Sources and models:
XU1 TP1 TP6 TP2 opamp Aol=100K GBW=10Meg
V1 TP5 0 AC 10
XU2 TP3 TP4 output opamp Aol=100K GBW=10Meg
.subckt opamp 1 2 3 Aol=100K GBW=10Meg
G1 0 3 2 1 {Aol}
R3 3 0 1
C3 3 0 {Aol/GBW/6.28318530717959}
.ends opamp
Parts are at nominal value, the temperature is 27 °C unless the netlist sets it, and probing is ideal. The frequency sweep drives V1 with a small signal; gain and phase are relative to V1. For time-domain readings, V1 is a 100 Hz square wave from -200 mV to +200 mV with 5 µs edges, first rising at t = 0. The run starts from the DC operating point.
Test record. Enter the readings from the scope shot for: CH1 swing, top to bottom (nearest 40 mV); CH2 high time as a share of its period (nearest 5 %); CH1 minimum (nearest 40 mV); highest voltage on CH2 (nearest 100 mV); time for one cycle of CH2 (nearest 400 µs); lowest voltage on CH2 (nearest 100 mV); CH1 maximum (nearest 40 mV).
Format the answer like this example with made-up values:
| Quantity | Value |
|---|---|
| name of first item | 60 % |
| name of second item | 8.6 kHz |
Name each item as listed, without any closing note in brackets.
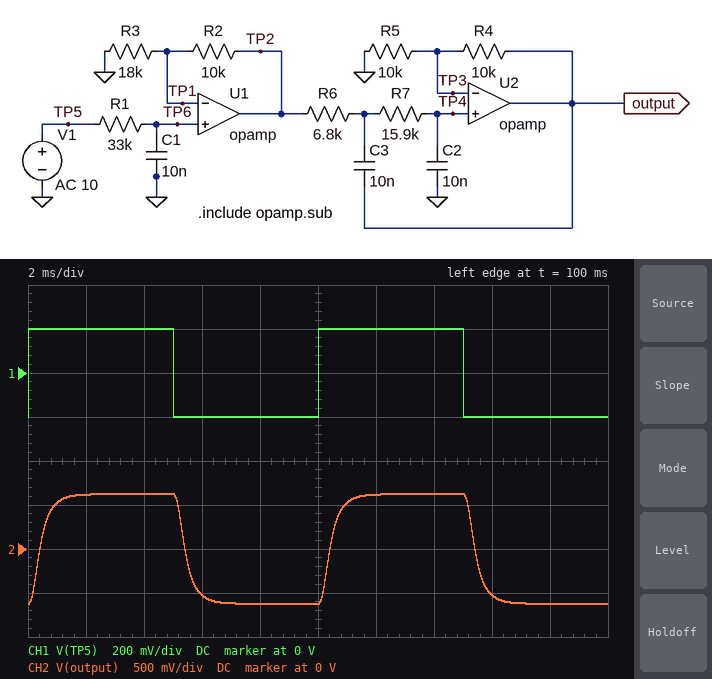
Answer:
| Quantity | Value |
|---|---|
| CH1 swing, top to bottom | 400 mV |
| CH2 high time as a share of its period | 50 % |
| CH1 minimum | -200 mV |
| highest voltage on CH2 | 600 mV |
| time for one cycle of CH2 | 10.0 ms |
| lowest voltage on CH2 | -600 mV |
| CH1 maximum | 200 mV |
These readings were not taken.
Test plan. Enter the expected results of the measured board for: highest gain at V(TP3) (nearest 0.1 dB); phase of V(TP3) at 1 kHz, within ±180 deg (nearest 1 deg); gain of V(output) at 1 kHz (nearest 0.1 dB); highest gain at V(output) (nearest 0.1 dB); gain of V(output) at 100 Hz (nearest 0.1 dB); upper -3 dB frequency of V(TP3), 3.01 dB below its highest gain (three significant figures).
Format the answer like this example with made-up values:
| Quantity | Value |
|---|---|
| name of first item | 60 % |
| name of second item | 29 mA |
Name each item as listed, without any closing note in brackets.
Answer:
| Quantity | Value |
|---|---|
| highest gain at V(TP3) | 3.8 dB |
| phase of V(TP3) at 1 kHz, within ±180 deg | -124 deg |
| gain of V(output) at 1 kHz | 1.4 dB |
| highest gain at V(output) | 9.9 dB |
| gain of V(output) at 100 Hz | 9.7 dB |
| upper -3 dB frequency of V(TP3), 3.01 dB below its highest gain | 464 Hz |
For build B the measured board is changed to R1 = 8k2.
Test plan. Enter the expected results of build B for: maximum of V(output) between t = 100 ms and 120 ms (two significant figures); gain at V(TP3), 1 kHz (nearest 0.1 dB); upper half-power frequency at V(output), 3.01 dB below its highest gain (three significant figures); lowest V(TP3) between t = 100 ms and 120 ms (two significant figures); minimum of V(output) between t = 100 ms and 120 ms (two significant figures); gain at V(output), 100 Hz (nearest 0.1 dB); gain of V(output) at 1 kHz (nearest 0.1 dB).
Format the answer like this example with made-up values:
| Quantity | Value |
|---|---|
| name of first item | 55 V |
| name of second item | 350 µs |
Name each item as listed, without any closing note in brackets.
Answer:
| Quantity | Value |
|---|---|
| maximum of V(output) between t = 100 ms and 120 ms | 640 mV |
| gain at V(TP3), 1 kHz | 1.6 dB |
| upper half-power frequency at V(output), 3.01 dB below its highest gain | 1.14 kHz |
| lowest V(TP3) between t = 100 ms and 120 ms | -320 mV |
| minimum of V(output) between t = 100 ms and 120 ms | -640 mV |
| gain at V(output), 100 Hz | 9.8 dB |
| gain of V(output) at 1 kHz | 7.6 dB |
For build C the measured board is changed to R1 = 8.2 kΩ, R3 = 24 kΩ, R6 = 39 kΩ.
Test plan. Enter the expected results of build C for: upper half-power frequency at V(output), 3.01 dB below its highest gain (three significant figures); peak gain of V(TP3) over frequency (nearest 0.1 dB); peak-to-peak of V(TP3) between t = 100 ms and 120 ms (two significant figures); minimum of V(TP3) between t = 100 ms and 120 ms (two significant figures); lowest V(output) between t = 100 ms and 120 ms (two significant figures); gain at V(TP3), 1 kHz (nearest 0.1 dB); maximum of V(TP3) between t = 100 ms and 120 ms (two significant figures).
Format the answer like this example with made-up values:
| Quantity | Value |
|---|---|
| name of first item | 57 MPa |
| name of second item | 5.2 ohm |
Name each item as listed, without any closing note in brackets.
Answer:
| Quantity | Value |
|---|---|
| upper half-power frequency at V(output), 3.01 dB below its highest gain | 747 Hz |
| peak gain of V(TP3) over frequency | 7.0 dB |
| peak-to-peak of V(TP3) between t = 100 ms and 120 ms | 940 mV |
| minimum of V(TP3) between t = 100 ms and 120 ms | -470 mV |
| lowest V(output) between t = 100 ms and 120 ms | -940 mV |
| gain at V(TP3), 1 kHz | -2.9 dB |
| maximum of V(TP3) between t = 100 ms and 120 ms | 470 mV |
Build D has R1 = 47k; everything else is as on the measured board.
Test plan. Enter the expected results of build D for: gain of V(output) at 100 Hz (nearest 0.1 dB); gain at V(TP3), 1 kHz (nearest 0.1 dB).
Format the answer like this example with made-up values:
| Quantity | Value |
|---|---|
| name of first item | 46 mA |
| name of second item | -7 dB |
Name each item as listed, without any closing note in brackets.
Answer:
| Quantity | Value |
|---|---|
| gain of V(output) at 100 Hz | 9.5 dB |
| gain at V(TP3), 1 kHz | -7.3 dB |
